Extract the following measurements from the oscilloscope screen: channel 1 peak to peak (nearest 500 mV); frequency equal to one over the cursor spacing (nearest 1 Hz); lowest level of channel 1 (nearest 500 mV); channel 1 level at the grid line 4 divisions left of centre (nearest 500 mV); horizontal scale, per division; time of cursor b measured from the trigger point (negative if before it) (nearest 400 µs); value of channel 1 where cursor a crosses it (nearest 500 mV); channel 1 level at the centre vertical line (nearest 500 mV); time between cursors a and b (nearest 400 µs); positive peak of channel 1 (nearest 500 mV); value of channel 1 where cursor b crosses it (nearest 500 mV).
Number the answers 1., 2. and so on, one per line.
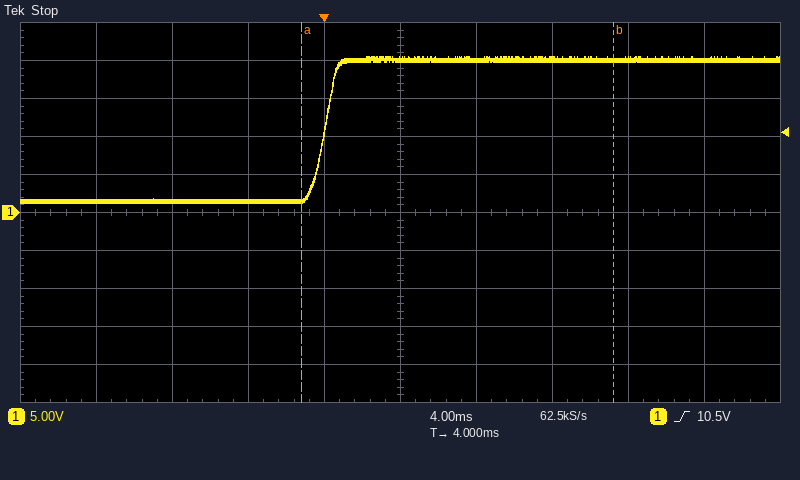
1. 19.0 V
2. 61 Hz
3. 1.5 V
4. 1.5 V
5. 4 ms
6. +15.2 ms
7. 1.5 V
8. 20.0 V
9. 16.4 ms
10. 20.5 V
11. 20.0 V
